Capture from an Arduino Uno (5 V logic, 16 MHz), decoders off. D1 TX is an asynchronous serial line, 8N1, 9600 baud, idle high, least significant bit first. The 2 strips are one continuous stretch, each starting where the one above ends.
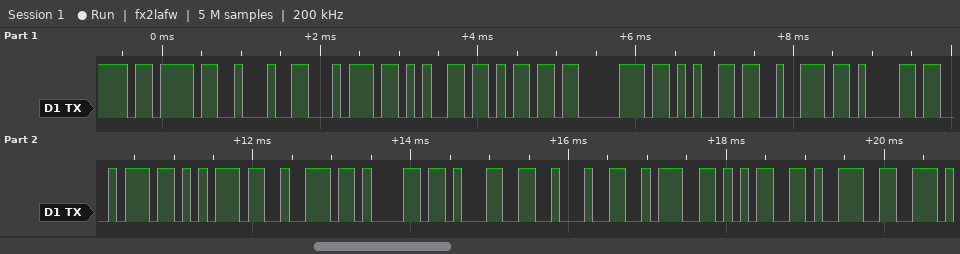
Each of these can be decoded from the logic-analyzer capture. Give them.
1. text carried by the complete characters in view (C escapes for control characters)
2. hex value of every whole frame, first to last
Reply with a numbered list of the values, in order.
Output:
1. "{\"temperatura1\":59"
2. 0x7B 0x22 0x74 0x65 0x6D 0x70 0x65 0x72 0x61 0x74 0x75 0x72 0x61 0x31 0x22 0x3A 0x35 0x39
